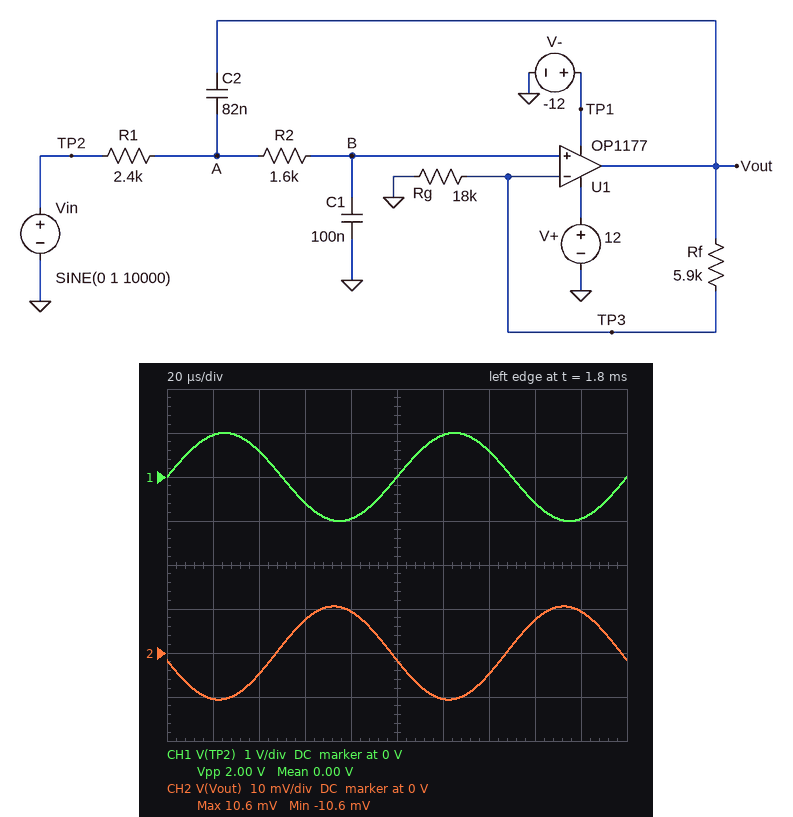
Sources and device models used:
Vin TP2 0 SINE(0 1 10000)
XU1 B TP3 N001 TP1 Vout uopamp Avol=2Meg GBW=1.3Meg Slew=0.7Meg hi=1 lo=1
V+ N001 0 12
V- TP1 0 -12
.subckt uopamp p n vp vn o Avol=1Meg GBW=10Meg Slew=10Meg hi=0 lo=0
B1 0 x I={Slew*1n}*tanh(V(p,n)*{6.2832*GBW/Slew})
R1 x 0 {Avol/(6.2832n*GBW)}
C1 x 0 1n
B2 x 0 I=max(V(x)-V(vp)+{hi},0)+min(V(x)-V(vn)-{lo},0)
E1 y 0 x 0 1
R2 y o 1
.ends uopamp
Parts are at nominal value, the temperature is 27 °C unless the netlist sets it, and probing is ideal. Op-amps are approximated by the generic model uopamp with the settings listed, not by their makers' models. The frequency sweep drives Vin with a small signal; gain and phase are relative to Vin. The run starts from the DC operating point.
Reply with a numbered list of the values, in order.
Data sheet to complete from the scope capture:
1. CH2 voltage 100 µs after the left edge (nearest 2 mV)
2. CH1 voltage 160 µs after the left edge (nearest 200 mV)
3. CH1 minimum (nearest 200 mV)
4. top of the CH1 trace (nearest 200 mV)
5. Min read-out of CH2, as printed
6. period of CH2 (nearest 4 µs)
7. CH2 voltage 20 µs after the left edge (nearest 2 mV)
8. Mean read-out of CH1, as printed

1. -2 mV
2. -600 mV
3. -1.0 V
4. 1.0 V
5. -10.6 mV
6. 100 µs
7. -10 mV
8. 0.00 V
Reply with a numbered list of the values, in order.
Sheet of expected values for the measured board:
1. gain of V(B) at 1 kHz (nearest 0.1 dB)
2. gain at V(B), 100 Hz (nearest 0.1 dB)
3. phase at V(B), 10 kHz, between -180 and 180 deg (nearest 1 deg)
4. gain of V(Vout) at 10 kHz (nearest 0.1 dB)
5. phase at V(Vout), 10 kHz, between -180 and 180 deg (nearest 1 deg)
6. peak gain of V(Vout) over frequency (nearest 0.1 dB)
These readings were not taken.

1. -6.5 dB
2. -0.1 dB
3. -170 deg
4. -39.5 dB
5. -171 deg
6. 2.5 dB
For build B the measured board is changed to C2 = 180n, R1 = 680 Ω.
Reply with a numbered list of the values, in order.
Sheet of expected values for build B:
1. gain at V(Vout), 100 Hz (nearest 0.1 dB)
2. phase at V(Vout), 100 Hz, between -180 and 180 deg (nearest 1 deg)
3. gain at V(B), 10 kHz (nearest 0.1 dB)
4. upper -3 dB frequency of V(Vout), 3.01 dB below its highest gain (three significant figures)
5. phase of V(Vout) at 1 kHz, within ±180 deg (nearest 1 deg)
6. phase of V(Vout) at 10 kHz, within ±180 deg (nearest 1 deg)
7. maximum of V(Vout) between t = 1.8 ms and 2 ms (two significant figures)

1. 2.5 dB
2. -7 deg
3. -37.8 dB
4. 1.19 kHz
5. -79 deg
6. -172 deg
7. 17 mV
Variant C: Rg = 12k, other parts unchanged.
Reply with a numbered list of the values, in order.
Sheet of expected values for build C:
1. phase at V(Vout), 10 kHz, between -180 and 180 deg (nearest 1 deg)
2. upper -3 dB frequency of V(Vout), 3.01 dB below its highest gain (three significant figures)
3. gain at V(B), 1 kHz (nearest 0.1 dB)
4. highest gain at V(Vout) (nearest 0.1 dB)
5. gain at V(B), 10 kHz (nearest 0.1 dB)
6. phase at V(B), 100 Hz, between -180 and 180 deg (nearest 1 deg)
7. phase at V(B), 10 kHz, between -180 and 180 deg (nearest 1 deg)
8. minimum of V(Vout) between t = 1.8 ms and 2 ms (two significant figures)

1. -172 deg
2. 718 Hz
3. -5.7 dB
4. 3.5 dB
5. -41.9 dB
6. -11 deg
7. -171 deg
8. -12 mV
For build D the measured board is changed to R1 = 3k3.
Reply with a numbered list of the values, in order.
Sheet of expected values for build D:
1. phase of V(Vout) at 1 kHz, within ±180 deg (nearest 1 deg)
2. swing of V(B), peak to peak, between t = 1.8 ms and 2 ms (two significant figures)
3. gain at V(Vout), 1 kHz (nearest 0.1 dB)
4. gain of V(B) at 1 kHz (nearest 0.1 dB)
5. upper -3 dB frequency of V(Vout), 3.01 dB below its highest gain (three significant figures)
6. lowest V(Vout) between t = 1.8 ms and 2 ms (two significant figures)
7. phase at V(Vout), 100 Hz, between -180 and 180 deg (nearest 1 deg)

1. -106 deg
2. 12 mV
3. -5.9 dB
4. -8.4 dB
5. 518 Hz
6. -7.7 mV
7. -14 deg
